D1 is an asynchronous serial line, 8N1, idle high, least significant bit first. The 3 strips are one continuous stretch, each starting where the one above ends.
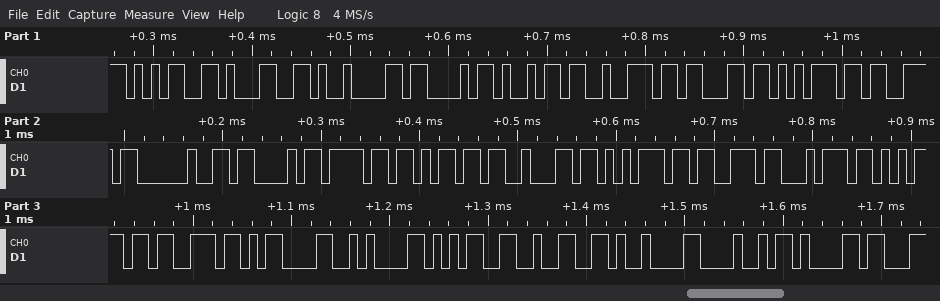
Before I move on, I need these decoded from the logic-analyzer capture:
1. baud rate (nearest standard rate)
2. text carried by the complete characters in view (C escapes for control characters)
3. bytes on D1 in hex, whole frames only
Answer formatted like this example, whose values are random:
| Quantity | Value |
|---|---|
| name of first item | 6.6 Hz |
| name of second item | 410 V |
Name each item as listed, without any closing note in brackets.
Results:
| Quantity | Value |
|---|---|
| baud rate | 115200 baud |
| text carried by the complete characters in view | "51\tCircus Combustus\r\n52\tHa" |
| bytes on D1 in hex, whole frames only | 35 31 09 43 69 72 63 75 73 20 43 6F 6D 62 75 73 74 75 73 0D 0A 35 32 09 48 61 |
